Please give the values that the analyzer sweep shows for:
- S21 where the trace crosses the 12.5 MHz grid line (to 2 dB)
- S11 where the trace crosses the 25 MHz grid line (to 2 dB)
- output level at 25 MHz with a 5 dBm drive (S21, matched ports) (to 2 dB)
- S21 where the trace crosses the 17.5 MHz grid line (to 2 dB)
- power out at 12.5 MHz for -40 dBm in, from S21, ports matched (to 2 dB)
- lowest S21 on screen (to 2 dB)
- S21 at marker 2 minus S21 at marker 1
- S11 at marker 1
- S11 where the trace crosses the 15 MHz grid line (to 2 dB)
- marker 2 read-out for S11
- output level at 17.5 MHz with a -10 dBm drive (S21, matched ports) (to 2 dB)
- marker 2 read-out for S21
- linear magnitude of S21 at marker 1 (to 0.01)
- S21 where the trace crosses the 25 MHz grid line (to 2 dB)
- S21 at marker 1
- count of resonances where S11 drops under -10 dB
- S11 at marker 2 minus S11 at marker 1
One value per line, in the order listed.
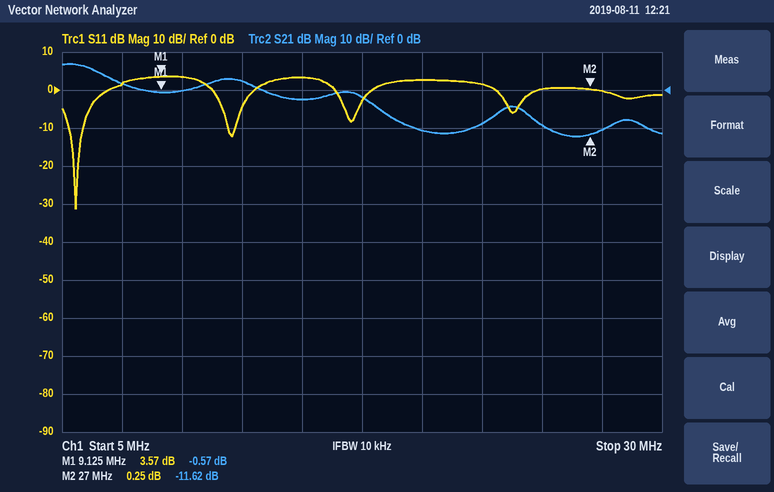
2 dB
0 dB
-4 dBm
-2 dB
-38 dBm
-12 dB
-11.05 dB
3.57 dB
4 dB
0.25 dB
-12 dBm
-11.62 dB
0.94
-10 dB
-0.57 dB
2
-3.32 dB
